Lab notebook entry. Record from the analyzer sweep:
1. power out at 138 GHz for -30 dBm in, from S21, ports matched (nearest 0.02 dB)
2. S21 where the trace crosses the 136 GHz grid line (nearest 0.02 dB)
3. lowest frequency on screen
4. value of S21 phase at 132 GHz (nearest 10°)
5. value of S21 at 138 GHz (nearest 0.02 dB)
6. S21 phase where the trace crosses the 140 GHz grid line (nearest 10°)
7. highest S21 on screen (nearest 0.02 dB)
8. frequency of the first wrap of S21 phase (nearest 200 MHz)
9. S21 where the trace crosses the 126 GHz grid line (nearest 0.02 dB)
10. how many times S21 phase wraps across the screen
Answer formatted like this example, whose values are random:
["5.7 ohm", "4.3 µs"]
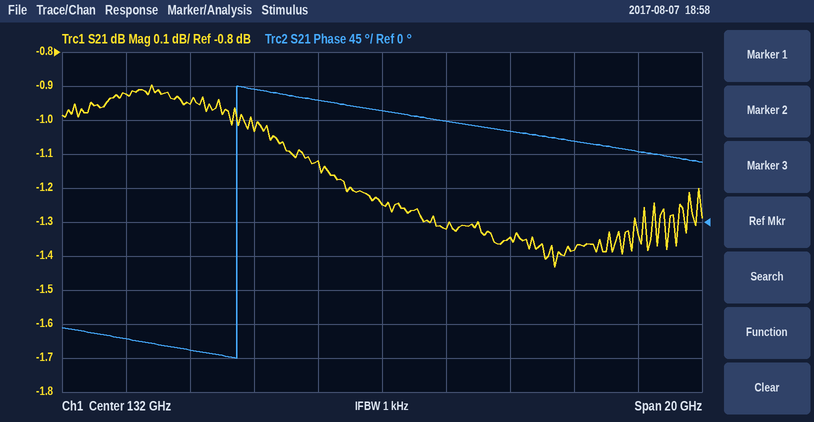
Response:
["-31.38 dBm", "-1.34 dB", "122 GHz", "150°", "-1.38 dB", "90°", "-0.90 dB", "127.4 GHz", "-0.96 dB", "1"]
